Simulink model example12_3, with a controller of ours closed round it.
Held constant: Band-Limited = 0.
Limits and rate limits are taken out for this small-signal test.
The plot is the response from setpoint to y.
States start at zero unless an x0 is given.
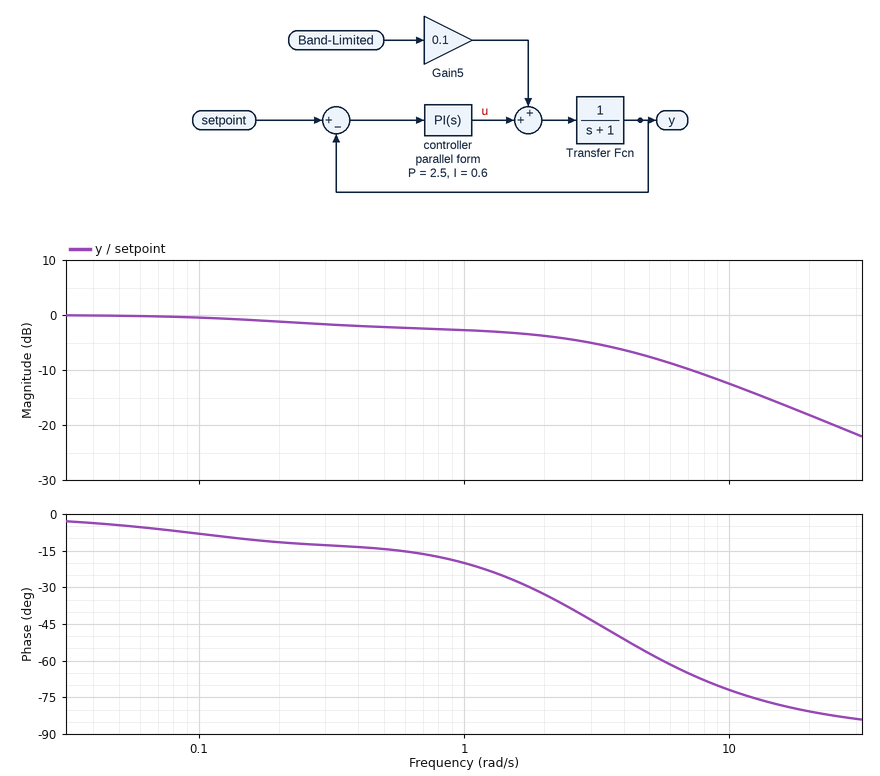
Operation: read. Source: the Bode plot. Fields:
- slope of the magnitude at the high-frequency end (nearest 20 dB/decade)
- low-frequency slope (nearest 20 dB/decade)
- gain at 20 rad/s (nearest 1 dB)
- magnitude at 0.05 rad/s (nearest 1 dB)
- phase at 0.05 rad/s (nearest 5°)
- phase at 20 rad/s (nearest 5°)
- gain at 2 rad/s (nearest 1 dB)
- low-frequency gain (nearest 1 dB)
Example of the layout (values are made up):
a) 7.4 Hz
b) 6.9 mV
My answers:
a) -20 dB/decade
b) 0 dB/decade
c) -18 dB
d) 0 dB
e) -5°
f) -80°
g) -4 dB
h) 0 dB
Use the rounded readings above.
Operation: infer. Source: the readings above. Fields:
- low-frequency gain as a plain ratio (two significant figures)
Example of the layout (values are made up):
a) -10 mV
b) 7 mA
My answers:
a) 1.0
